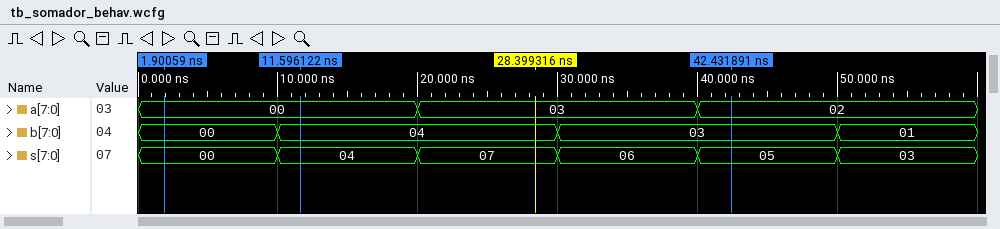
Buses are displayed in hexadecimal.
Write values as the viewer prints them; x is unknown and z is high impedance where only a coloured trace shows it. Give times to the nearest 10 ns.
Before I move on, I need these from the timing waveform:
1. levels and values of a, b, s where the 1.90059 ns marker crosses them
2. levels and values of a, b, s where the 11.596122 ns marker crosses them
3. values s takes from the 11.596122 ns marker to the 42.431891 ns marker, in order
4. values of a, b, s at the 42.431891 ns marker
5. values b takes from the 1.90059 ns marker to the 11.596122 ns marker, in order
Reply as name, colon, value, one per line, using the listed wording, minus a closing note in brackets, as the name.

levels and values of a, b, s where the 1.90059 ns marker crosses them: a=00, b=00, s=00
levels and values of a, b, s where the 11.596122 ns marker crosses them: a=00, b=04, s=04
values s takes from the 11.596122 ns marker to the 42.431891 ns marker, in order: 04, 07, 06, 05
values of a, b, s at the 42.431891 ns marker: a=02, b=03, s=05
values b takes from the 1.90059 ns marker to the 11.596122 ns marker, in order: 00, 04
